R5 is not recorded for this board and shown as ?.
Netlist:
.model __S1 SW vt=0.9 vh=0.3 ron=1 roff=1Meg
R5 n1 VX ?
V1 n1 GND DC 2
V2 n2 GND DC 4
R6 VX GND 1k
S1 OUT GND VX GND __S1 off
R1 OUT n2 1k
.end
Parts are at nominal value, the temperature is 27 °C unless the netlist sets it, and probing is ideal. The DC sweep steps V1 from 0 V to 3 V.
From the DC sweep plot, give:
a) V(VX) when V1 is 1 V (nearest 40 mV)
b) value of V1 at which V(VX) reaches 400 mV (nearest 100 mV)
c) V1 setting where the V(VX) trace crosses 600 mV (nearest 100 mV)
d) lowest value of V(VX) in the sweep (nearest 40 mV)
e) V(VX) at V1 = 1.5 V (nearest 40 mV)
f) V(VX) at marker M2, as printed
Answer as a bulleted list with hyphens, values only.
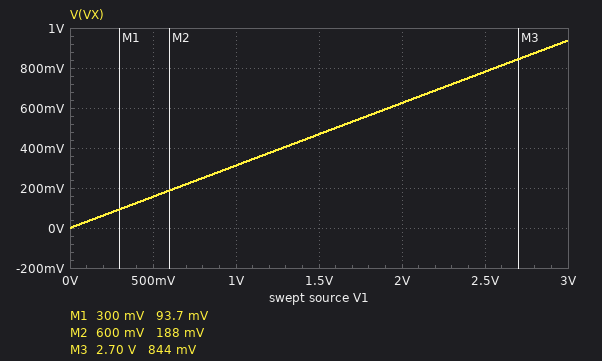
- 320 mV
- 1.3 V
- 1.9 V
- 0 V
- 480 mV
- 188 mV
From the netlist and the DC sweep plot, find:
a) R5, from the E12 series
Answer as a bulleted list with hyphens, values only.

- 2.2 kΩ
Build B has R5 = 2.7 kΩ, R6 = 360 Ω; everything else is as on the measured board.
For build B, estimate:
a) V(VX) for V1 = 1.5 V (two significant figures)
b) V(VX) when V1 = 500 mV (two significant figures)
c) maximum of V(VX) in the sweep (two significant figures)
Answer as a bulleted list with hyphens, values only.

- 180 mV
- 59 mV
- 350 mV
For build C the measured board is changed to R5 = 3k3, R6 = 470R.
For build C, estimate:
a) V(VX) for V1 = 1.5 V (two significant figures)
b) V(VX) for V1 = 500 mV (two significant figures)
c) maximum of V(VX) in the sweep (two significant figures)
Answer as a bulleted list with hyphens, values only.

- 190 mV
- 62 mV
- 370 mV
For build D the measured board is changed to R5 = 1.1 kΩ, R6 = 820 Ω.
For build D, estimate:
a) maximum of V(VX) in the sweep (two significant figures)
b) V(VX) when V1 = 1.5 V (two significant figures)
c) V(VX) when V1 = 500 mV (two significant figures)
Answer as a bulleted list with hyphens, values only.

- 1.3 V
- 640 mV
- 210 mV
